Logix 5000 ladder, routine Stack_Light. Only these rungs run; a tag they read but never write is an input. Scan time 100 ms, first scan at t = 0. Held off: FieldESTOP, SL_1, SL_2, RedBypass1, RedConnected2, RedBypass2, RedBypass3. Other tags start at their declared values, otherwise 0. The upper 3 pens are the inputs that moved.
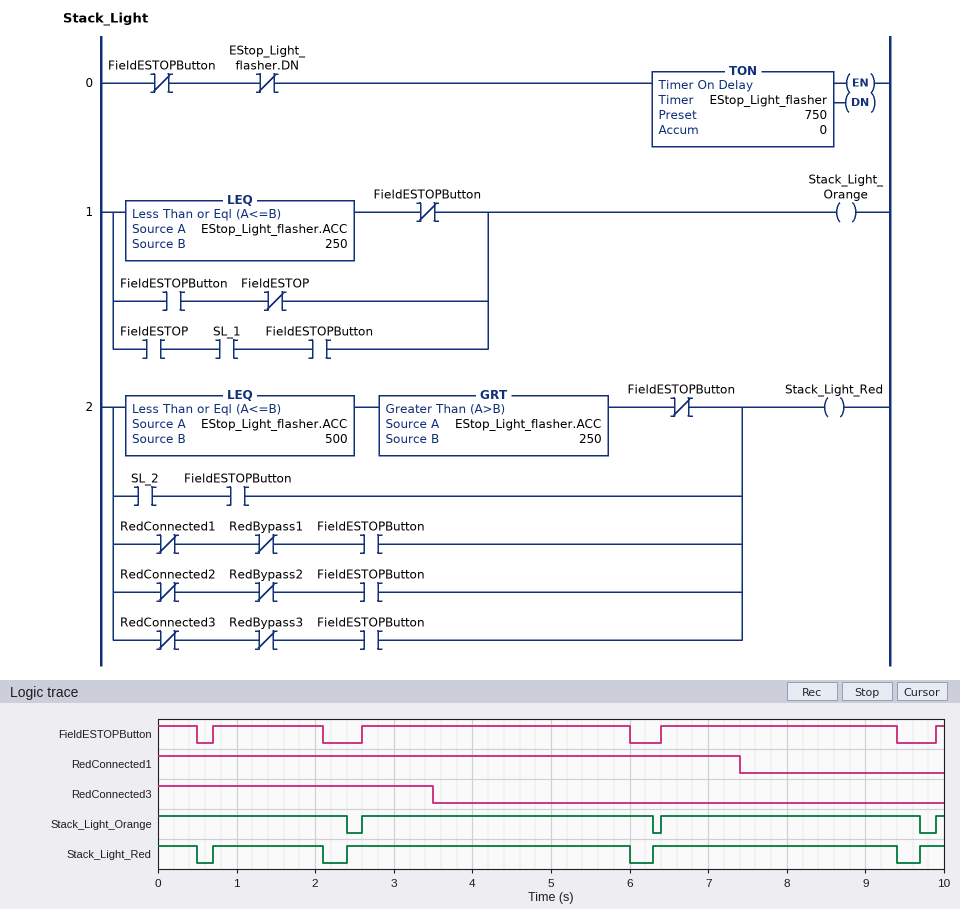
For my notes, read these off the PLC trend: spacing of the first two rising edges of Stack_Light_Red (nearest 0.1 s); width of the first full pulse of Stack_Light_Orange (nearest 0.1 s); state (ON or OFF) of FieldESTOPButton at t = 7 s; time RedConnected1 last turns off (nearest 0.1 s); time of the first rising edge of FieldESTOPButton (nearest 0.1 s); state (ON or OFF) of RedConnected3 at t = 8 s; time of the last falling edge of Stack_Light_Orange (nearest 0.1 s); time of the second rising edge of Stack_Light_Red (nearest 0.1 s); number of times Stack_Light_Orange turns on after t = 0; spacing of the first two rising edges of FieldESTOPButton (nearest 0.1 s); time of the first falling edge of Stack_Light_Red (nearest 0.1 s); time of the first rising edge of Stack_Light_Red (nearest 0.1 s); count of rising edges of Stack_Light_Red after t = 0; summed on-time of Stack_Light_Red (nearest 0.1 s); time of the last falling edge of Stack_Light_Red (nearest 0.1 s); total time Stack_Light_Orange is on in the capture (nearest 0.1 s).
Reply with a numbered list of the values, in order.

1. 1.7 s
2. 3.7 s
3. ON
4. 7.4 s
5. 0.7 s
6. OFF
7. 9.7 s
8. 2.4 s
9. 3
10. 1.9 s
11. 0.5 s
12. 0.7 s
13. 4
14. 8.9 s
15. 9.4 s
16. 9.5 s
